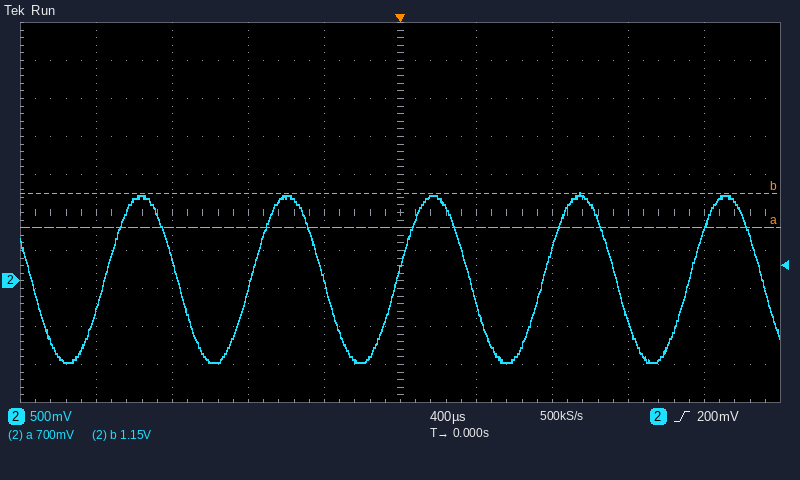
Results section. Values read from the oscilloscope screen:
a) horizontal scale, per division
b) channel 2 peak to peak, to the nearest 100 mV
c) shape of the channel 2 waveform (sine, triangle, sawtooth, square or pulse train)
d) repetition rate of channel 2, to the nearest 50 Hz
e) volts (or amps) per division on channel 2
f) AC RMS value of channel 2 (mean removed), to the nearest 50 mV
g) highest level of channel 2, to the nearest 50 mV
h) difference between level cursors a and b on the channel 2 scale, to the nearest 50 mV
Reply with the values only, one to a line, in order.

400 µs
2.20 V
sine
1.30 kHz
500 mV
800 mV
1.15 V
450 mV
